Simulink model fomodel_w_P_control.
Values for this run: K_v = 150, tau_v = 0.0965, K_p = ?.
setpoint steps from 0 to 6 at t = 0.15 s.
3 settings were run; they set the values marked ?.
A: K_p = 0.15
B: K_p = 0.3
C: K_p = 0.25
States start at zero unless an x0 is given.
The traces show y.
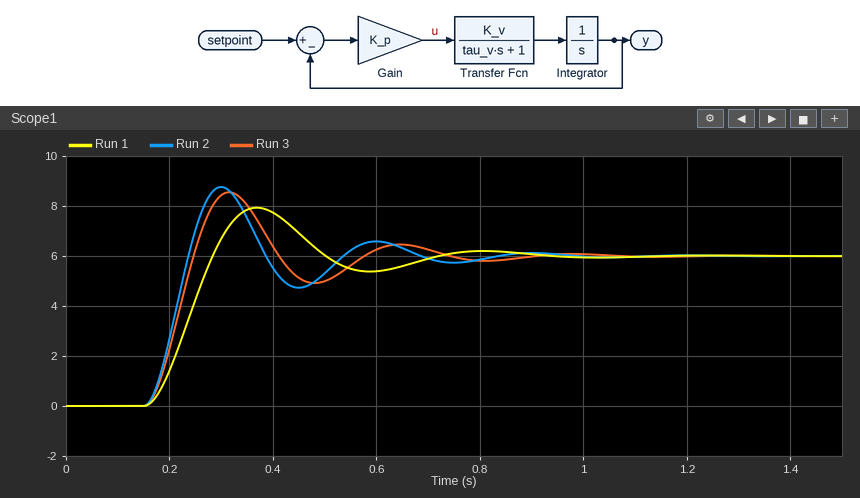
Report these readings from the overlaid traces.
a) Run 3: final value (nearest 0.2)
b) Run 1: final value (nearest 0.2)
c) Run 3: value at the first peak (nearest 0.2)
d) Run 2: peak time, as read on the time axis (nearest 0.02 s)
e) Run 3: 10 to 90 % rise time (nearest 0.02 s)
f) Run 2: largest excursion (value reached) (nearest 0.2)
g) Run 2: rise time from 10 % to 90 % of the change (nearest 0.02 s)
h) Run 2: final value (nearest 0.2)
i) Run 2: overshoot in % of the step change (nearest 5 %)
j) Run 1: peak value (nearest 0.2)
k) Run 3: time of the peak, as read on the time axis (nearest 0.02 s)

6.0
6.0
8.6
0.30 s
0.06 s
8.8
0.06 s
6.0
45 %
8.0
0.32 s
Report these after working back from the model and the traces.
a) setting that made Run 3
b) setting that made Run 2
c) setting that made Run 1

C
B
A
